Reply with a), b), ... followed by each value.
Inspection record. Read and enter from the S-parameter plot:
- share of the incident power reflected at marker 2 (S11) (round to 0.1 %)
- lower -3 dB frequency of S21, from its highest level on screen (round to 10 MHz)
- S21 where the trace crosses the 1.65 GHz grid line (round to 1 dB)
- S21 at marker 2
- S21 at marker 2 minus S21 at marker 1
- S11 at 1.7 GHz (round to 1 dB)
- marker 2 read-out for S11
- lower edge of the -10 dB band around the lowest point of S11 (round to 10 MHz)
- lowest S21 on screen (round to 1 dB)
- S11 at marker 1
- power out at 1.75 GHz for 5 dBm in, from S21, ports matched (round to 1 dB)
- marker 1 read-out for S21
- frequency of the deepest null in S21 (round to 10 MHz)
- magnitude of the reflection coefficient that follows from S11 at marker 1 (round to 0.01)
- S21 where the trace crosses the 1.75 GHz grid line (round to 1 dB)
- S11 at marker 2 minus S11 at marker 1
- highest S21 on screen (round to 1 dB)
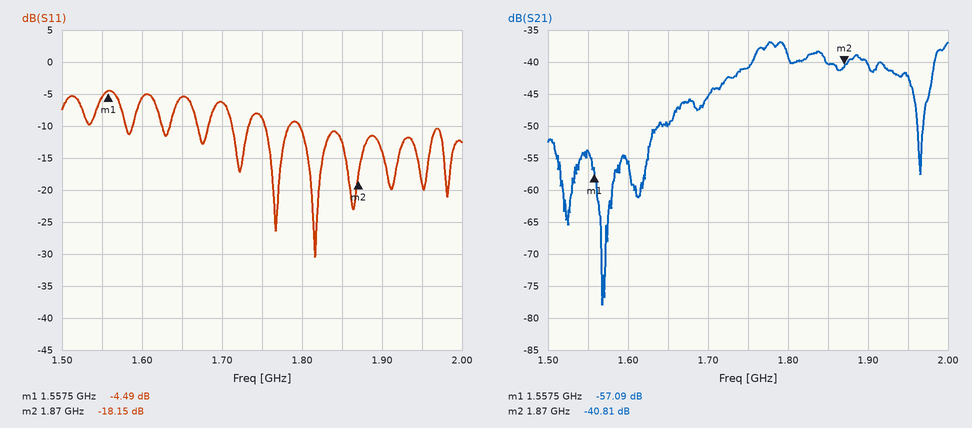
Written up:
a) 1.5 %
b) 1.76 GHz
c) -50 dB
d) -40.81 dB
e) 16.28 dB
f) -6 dB
g) -18.15 dB
h) 1.80 GHz
i) -78 dB
j) -4.49 dB
k) -36 dBm
l) -57.09 dB
m) 1.57 GHz
n) 0.60
o) -41 dB
p) -13.66 dB
q) -37 dB
